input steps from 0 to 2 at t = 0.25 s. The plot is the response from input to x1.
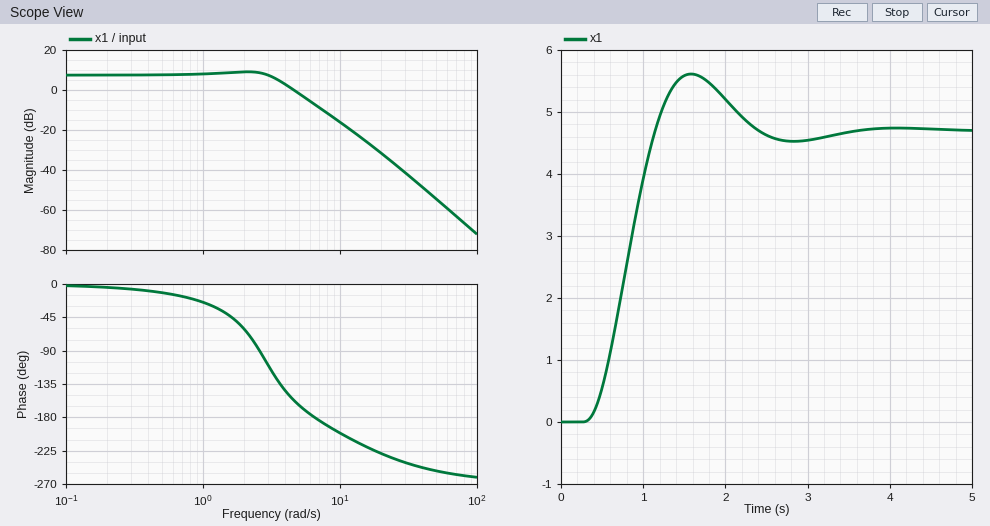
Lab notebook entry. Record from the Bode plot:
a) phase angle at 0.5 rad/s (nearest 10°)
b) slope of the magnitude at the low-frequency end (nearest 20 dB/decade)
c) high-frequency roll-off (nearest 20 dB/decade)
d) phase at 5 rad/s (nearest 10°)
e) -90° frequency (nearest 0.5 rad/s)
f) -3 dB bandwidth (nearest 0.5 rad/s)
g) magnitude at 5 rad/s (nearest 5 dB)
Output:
-10°
0 dB/decade
-60 dB/decade
-160°
2.5 rad/s
3.5 rad/s
0 dB
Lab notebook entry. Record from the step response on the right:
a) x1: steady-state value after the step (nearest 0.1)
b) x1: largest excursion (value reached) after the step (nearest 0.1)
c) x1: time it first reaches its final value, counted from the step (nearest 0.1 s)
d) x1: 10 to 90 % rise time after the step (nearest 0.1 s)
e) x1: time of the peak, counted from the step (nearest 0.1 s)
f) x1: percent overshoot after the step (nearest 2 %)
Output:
4.7
5.6
0.9 s
0.6 s
1.3 s
20 %
